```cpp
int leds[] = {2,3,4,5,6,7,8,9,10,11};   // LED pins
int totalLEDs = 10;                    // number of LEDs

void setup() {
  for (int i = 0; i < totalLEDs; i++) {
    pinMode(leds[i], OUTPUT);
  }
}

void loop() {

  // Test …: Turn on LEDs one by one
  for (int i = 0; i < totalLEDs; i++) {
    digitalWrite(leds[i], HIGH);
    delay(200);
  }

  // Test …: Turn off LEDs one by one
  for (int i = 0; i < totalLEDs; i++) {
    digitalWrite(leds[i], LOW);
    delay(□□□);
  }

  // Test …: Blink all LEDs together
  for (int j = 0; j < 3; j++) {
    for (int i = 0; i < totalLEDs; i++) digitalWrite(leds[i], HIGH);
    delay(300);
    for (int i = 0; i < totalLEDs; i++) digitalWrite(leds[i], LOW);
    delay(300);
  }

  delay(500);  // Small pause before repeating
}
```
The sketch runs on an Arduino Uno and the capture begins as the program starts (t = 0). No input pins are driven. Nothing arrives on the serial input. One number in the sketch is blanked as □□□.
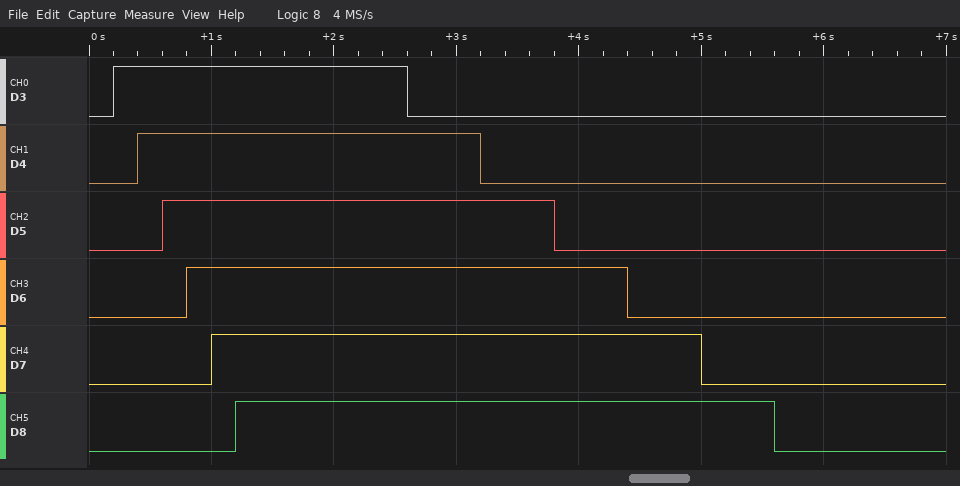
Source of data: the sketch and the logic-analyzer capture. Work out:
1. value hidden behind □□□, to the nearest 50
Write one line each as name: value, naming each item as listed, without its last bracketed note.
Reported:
value hidden behind □□□, to the nearest 50: 600
